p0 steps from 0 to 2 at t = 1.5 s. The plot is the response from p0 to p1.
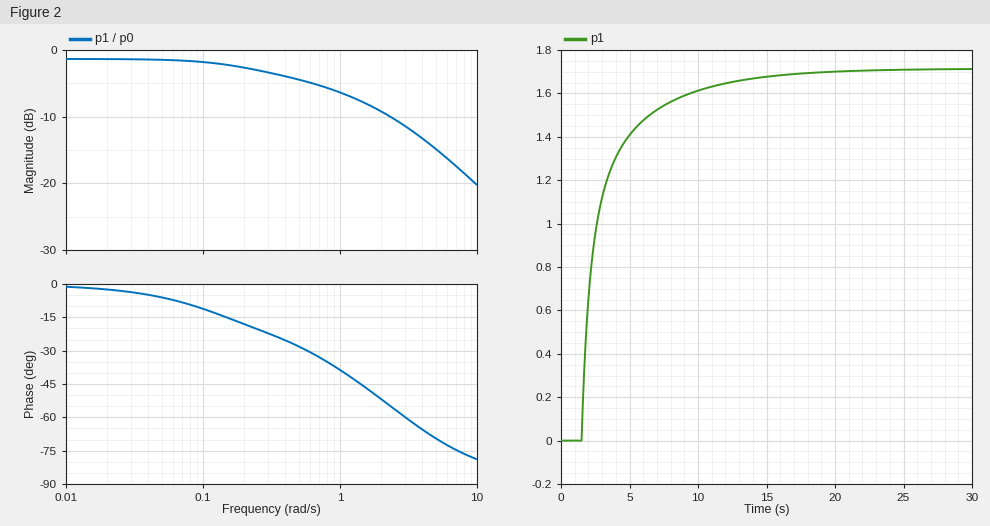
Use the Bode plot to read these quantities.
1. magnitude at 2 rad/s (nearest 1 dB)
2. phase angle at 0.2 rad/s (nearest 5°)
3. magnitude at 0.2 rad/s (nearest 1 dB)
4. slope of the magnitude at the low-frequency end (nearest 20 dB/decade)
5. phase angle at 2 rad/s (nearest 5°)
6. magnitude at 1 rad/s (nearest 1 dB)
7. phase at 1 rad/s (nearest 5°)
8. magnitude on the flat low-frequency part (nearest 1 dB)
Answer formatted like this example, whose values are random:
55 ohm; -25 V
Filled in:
-9 dB; -20°; -3 dB; 0 dB/decade; -50°; -6 dB; -40°; -1 dB
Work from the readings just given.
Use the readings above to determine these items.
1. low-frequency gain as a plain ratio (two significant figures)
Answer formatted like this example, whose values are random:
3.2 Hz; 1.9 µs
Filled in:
0.89
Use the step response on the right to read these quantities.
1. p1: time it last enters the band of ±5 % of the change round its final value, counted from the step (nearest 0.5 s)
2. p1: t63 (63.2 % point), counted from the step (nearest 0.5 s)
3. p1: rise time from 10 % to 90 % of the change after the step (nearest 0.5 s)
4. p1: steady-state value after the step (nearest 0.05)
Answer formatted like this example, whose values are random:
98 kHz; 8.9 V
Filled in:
9.5 s; 1.5 s; 6.0 s; 1.70
